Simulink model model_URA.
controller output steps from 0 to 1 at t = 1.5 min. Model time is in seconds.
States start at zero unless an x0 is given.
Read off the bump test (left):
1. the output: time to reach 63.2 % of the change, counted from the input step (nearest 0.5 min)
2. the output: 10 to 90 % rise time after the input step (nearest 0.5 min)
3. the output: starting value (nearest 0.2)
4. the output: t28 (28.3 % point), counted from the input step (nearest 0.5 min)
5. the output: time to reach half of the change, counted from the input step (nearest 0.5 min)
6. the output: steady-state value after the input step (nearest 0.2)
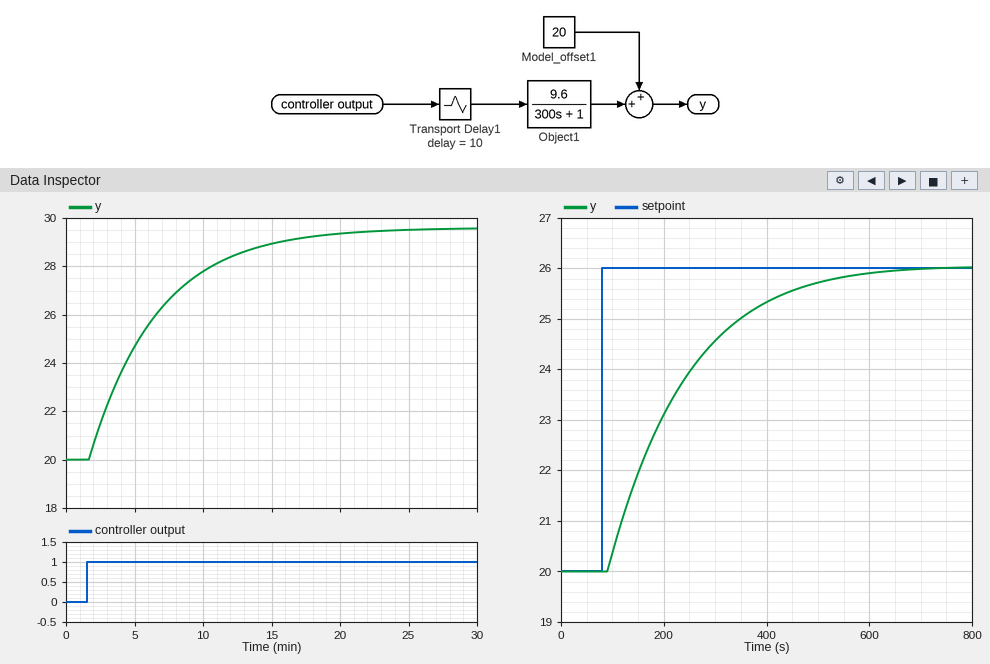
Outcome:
5.0 min
11.0 min
20.0
2.0 min
3.5 min
29.6
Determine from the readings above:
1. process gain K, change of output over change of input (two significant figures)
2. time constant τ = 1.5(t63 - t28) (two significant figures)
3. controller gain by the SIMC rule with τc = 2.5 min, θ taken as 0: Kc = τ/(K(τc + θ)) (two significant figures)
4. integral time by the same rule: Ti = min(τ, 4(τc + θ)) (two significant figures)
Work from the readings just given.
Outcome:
9.6
4.5 min
0.19
4.5 min
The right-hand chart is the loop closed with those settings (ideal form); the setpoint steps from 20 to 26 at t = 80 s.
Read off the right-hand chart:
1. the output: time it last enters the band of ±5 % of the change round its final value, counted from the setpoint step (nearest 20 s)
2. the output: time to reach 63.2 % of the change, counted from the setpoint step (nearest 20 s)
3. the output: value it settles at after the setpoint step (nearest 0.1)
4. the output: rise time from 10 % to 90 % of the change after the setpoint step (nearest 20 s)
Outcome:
420 s
160 s
26.0
300 s
